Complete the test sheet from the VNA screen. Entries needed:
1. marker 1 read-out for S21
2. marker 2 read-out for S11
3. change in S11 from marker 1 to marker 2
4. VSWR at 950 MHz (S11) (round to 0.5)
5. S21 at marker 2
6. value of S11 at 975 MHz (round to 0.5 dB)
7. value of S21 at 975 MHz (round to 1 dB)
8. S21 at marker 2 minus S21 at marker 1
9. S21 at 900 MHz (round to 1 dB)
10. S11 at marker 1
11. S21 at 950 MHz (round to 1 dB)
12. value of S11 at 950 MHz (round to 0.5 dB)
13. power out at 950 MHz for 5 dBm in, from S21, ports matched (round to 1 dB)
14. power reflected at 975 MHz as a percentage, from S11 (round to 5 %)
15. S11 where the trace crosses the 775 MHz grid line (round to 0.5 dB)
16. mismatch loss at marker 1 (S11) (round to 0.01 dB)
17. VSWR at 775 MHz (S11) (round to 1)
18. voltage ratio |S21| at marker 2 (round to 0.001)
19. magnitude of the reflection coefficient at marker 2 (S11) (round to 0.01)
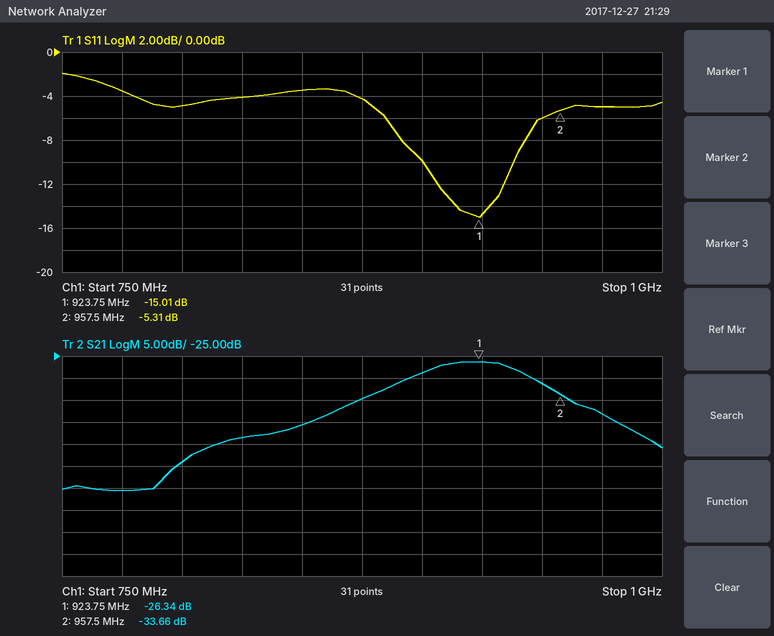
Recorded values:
-26.34 dB
-5.31 dB
9.70 dB
3.0
-33.66 dB
-5.0 dB
-38 dB
-7.32 dB
-29 dB
-15.01 dB
-31 dB
-6.0 dB
-26 dBm
30 %
-3.5 dB
0.14 dB
5
0.021
0.54
